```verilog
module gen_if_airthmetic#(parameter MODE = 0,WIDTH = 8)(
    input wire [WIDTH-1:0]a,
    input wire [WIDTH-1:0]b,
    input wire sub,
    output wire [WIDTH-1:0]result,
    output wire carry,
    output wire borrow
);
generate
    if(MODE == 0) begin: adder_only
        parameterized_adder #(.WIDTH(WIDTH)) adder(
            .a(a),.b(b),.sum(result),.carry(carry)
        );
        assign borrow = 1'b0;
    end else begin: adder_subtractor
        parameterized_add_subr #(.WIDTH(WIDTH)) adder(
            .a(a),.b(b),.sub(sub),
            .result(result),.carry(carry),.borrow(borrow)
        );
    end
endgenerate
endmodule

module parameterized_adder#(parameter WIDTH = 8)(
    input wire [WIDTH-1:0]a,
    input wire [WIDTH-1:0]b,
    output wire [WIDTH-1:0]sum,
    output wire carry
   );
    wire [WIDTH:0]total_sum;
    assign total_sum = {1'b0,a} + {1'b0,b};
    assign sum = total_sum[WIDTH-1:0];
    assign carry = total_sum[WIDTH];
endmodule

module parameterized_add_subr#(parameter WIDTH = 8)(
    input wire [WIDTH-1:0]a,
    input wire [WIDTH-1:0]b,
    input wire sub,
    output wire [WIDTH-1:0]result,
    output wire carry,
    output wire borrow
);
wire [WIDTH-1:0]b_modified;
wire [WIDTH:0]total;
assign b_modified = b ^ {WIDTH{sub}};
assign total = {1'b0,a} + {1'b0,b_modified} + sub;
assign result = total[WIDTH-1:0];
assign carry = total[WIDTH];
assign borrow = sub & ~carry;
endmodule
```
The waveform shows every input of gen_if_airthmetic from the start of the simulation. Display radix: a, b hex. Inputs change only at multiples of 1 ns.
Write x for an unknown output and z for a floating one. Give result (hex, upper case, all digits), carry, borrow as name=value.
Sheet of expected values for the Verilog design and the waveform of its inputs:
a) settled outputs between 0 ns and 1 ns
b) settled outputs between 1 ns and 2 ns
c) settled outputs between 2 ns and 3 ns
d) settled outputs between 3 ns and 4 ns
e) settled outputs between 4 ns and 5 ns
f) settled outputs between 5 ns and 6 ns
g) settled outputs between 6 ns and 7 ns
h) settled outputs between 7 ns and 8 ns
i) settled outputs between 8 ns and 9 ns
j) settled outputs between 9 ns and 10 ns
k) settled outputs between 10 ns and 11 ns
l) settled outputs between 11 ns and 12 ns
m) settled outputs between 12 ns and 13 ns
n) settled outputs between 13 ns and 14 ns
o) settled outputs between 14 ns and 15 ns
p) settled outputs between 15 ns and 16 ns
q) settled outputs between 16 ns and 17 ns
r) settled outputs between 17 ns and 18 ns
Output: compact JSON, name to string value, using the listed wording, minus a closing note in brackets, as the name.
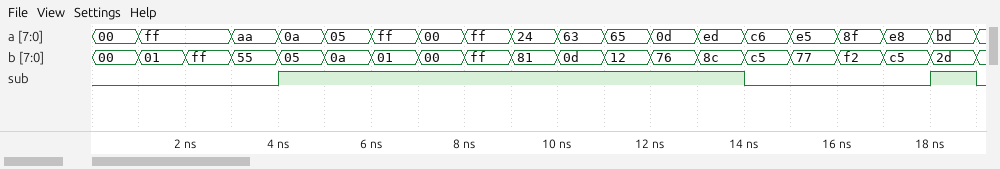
{"settled outputs between 0 ns and 1 ns": "result=00, carry=0, borrow=0", "settled outputs between 1 ns and 2 ns": "result=00, carry=1, borrow=0", "settled outputs between 2 ns and 3 ns": "result=FE, carry=1, borrow=0", "settled outputs between 3 ns and 4 ns": "result=FF, carry=0, borrow=0", "settled outputs between 4 ns and 5 ns": "result=0F, carry=0, borrow=0", "settled outputs between 5 ns and 6 ns": "result=0F, carry=0, borrow=0", "settled outputs between 6 ns and 7 ns": "result=00, carry=1, borrow=0", "settled outputs between 7 ns and 8 ns": "result=00, carry=0, borrow=0", "settled outputs between 8 ns and 9 ns": "result=FE, carry=1, borrow=0", "settled outputs between 9 ns and 10 ns": "result=A5, carry=0, borrow=0", "settled outputs between 10 ns and 11 ns": "result=70, carry=0, borrow=0", "settled outputs between 11 ns and 12 ns": "result=77, carry=0, borrow=0", "settled outputs between 12 ns and 13 ns": "result=83, carry=0, borrow=0", "settled outputs between 13 ns and 14 ns": "result=79, carry=1, borrow=0", "settled outputs between 14 ns and 15 ns": "result=8B, carry=1, borrow=0", "settled outputs between 15 ns and 16 ns": "result=5C, carry=1, borrow=0", "settled outputs between 16 ns and 17 ns": "result=81, carry=1, borrow=0", "settled outputs between 17 ns and 18 ns": "result=AD, carry=1, borrow=0"}
